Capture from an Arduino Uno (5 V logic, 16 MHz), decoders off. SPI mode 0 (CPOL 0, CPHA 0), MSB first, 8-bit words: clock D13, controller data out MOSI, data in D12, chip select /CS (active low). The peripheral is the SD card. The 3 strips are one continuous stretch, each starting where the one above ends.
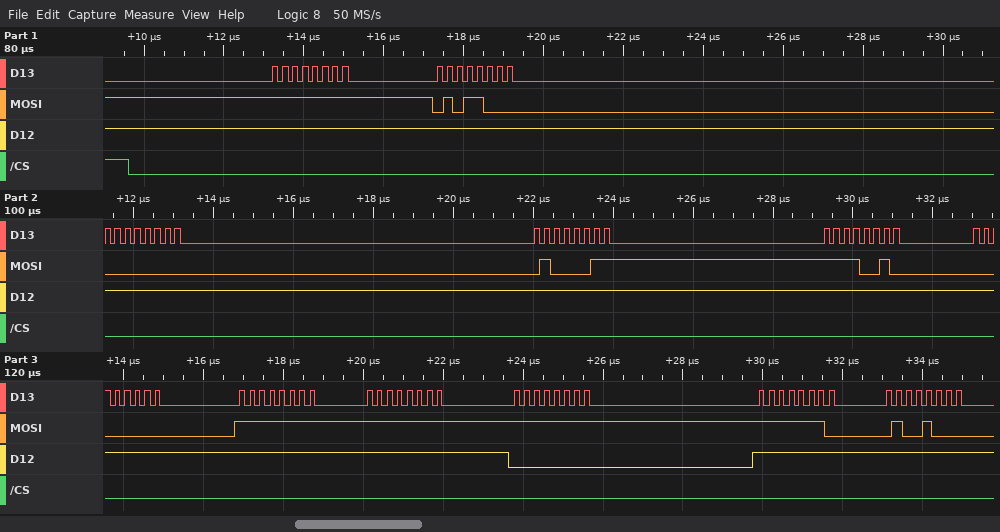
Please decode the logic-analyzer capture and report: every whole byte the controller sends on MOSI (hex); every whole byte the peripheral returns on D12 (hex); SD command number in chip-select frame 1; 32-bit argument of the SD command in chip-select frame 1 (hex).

0xFF 0x58 0x00 0x43 0xF2 0x00 0xFF 0xFF 0xFF 0xFE 0x48
0xFF 0xFF 0xFF 0xFF 0xFF 0xFF 0xFF 0xFF 0x00 0xFF 0xFF
CMD24
0x0043F200
